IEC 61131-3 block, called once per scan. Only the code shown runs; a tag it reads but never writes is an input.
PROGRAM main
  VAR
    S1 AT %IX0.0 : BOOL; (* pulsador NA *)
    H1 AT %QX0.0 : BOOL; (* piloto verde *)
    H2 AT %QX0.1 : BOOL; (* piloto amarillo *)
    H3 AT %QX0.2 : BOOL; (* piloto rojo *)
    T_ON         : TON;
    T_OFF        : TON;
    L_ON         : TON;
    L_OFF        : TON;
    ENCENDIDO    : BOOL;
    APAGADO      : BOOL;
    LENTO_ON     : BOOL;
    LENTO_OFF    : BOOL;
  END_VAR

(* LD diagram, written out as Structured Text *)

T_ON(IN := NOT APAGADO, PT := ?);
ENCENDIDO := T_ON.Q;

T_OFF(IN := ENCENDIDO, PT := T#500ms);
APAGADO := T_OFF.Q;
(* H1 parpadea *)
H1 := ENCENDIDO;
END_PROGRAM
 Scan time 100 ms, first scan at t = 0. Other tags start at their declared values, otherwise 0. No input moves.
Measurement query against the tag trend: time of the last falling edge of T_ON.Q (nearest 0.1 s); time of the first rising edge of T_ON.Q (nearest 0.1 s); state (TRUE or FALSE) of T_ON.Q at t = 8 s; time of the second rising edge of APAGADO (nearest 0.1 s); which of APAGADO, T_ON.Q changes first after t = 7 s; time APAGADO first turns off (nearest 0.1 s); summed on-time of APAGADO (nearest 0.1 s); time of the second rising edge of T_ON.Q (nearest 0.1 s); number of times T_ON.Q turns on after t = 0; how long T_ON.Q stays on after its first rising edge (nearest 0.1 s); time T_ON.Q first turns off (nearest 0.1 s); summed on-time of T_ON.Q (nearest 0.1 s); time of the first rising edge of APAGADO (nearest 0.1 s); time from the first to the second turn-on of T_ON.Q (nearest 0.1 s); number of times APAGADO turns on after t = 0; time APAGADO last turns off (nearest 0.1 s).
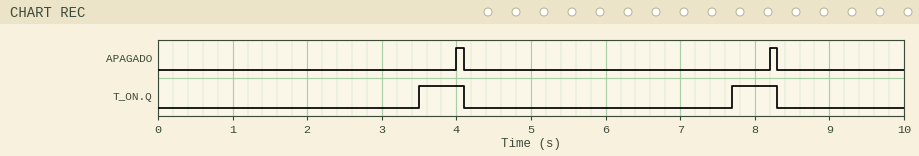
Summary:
8.3 s
3.5 s
TRUE
8.2 s
T_ON.Q
4.1 s
0.2 s
7.7 s
2
0.6 s
4.1 s
1.2 s
4.0 s
4.2 s
2
8.3 s
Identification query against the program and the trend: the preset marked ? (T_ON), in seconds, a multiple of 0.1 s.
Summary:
3.5 s
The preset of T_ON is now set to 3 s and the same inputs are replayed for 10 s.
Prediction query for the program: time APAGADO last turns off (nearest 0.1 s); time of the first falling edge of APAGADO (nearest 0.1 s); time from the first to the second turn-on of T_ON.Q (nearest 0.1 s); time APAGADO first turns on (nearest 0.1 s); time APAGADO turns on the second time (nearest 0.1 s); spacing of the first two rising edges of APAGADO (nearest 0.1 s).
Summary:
7.3 s
3.6 s
3.7 s
3.5 s
7.2 s
3.7 s
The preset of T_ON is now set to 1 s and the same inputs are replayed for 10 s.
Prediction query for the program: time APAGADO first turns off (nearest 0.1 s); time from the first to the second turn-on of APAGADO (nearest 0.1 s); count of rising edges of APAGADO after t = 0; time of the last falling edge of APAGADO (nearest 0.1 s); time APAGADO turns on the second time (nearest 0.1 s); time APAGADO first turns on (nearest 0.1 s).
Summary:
1.6 s
1.7 s
5
8.4 s
3.2 s
1.5 s
